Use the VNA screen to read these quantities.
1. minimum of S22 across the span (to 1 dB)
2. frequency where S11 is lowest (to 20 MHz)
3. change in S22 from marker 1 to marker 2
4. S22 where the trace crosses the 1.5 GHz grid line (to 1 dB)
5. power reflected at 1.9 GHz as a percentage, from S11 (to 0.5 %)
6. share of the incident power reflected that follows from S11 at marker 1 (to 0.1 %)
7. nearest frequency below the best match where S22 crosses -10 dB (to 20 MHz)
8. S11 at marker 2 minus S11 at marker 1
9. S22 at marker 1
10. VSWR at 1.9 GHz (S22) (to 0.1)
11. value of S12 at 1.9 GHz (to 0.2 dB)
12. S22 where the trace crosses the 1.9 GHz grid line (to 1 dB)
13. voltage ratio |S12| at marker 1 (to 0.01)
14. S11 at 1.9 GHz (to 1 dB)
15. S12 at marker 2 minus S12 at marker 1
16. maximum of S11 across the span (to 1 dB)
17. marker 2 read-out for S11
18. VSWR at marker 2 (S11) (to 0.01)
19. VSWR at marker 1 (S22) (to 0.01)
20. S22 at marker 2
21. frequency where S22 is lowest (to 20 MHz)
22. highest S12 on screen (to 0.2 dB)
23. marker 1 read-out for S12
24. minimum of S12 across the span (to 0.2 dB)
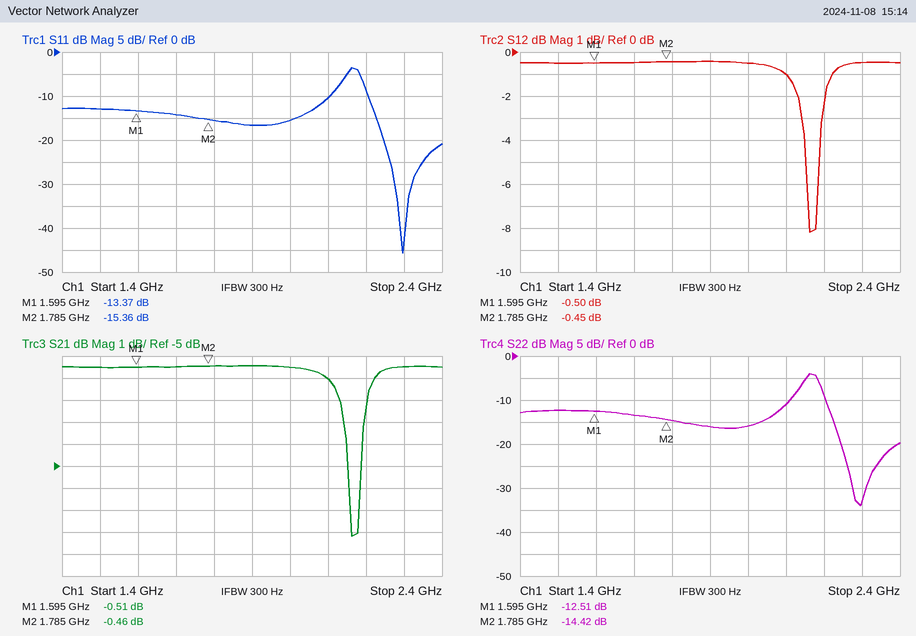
-34 dB
2.30 GHz
-1.91 dB
-12 dB
2.0 %
4.6 %
2.20 GHz
-1.99 dB
-12.51 dB
1.4
-0.4 dB
-16 dB
0.94
-17 dB
0.05 dB
-4 dB
-15.36 dB
1.41
1.62
-14.42 dB
2.30 GHz
-0.4 dB
-0.50 dB
-8.2 dB
